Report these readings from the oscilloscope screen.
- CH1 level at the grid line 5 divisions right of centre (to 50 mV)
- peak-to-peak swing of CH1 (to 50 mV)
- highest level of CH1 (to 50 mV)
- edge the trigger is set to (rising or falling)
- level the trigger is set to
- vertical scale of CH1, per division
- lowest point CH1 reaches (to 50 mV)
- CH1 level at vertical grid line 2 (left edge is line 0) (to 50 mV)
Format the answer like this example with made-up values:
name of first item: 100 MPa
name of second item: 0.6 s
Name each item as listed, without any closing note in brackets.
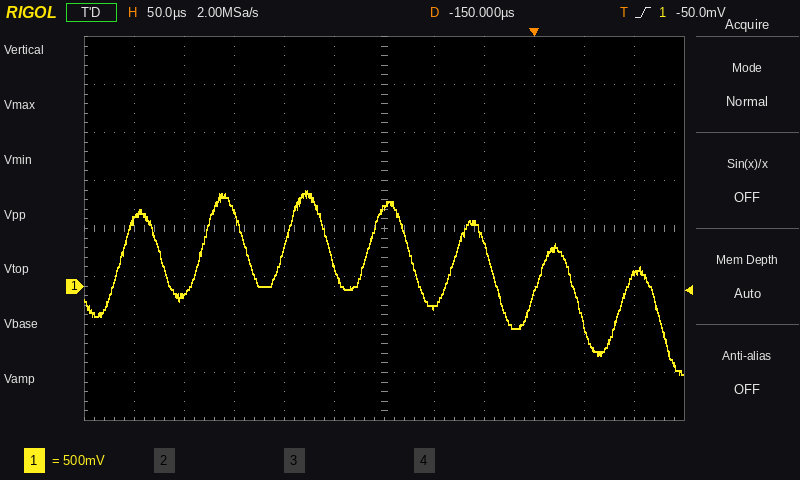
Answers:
CH1 level at the grid line 5 divisions right of centre: 100 mV
peak-to-peak swing of CH1: 1.90 V
highest level of CH1: 1.00 V
edge the trigger is set to: rising
level the trigger is set to: -50.0 mV
vertical scale of CH1, per division: 500 mV
lowest point CH1 reaches: -900 mV
CH1 level at vertical grid line 2 (left edge is line 0): -100 mV
